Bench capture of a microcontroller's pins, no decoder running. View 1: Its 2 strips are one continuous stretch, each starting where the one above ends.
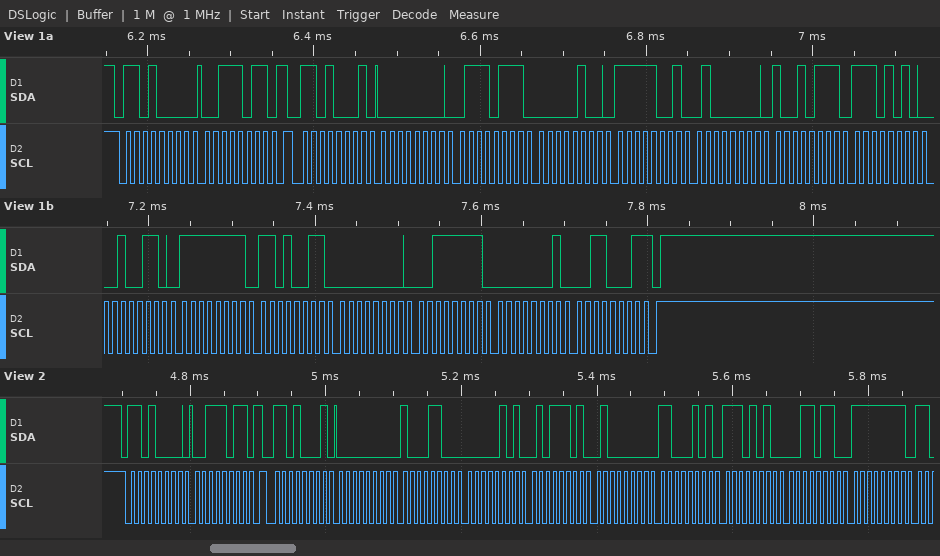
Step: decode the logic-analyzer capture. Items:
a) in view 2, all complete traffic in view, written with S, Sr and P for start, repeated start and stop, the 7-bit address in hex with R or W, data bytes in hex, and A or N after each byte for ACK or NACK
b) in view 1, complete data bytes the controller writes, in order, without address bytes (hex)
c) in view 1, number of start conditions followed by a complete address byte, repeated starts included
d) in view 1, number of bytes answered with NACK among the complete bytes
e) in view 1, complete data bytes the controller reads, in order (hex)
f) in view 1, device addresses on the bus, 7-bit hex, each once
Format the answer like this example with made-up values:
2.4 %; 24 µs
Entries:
S 68W A 3B A Sr 68R A 00 A 8C A 05 A 5D A 40 A C5 A EA A 36 A FF A; 3B; 2; 1; 00 77 04 F9 40 97 EA 26 FF D3 00 3F 01 31; 0x68
